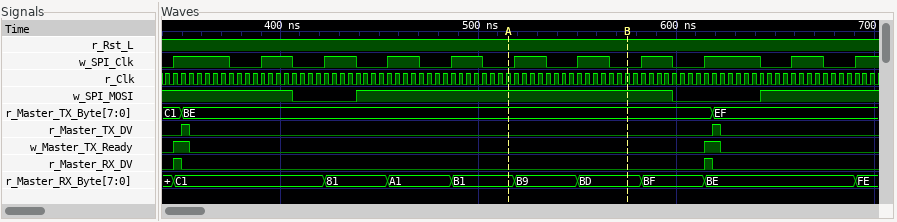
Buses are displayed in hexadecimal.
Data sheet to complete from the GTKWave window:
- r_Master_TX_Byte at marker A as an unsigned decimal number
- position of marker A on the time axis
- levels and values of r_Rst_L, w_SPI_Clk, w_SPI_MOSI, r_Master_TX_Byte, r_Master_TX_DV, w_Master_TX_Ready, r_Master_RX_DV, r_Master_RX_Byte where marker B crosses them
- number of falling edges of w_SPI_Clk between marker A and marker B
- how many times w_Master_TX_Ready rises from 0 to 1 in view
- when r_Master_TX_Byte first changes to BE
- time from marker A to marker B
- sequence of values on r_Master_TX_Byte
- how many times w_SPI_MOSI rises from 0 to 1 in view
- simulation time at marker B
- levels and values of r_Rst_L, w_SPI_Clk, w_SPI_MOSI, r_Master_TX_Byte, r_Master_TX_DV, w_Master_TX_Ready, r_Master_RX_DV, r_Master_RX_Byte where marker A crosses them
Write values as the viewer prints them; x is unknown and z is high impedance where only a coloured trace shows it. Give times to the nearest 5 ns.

190
515 ns
r_Rst_L=1, w_SPI_Clk=0, w_SPI_MOSI=1, r_Master_TX_Byte=BE, r_Master_TX_DV=0, w_Master_TX_Ready=0, r_Master_RX_DV=0, r_Master_RX_Byte=BD
2
2
350 ns
60 ns
C1, BE, EF
2
575 ns
r_Rst_L=1, w_SPI_Clk=0, w_SPI_MOSI=1, r_Master_TX_Byte=BE, r_Master_TX_DV=0, w_Master_TX_Ready=0, r_Master_RX_DV=0, r_Master_RX_Byte=B1
